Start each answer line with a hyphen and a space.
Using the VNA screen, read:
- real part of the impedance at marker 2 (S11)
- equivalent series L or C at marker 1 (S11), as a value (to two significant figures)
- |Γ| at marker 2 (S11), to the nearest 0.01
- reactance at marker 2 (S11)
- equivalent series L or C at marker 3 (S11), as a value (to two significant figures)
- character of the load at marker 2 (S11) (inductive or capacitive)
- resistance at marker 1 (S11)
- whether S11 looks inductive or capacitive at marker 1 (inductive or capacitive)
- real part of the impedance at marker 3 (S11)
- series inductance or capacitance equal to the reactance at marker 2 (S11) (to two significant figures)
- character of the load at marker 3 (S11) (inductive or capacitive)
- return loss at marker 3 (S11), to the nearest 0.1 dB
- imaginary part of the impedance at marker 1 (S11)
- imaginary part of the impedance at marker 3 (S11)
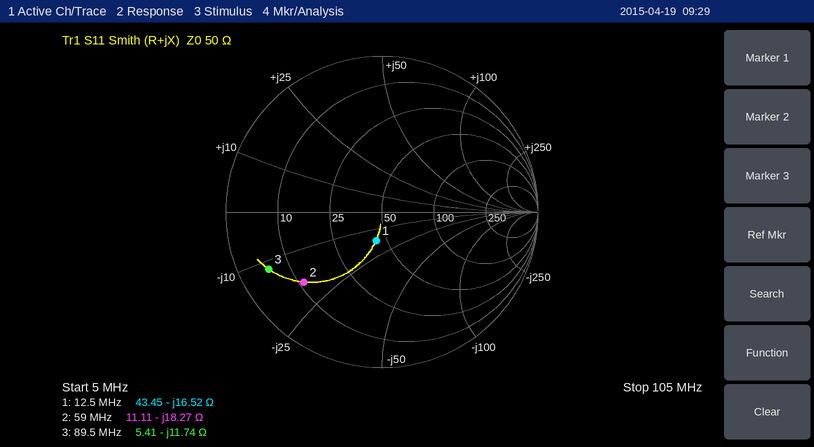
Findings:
- 11.11 Ω
- 770 pF
- 0.67
- -18.27 Ω
- 150 pF
- capacitive
- 43.45 Ω
- capacitive
- 5.41 Ω
- 150 pF
- capacitive
- 1.8 dB
- -16.52 Ω
- -11.74 Ω
